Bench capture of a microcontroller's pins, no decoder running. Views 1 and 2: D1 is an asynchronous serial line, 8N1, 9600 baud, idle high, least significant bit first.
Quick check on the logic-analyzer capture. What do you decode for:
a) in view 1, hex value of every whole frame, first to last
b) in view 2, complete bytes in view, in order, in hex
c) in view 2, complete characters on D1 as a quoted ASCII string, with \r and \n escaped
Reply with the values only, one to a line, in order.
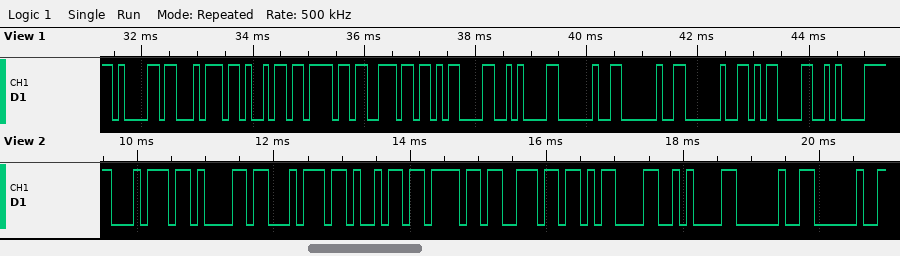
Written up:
61 74 69 6F 6E 0D 0A 20 20 20 0D 0A
74 61 74 69 6F 6E 0D 0A 20 20
"tation\r\n  "
